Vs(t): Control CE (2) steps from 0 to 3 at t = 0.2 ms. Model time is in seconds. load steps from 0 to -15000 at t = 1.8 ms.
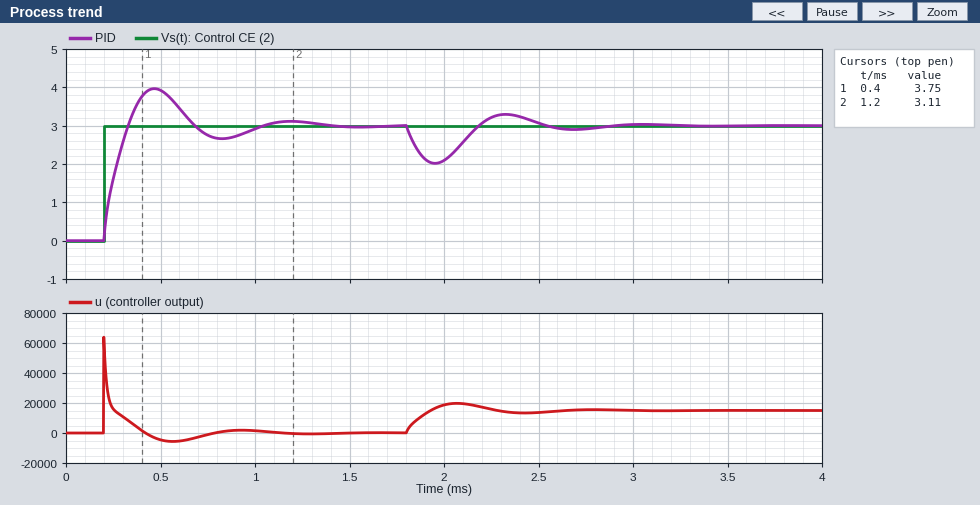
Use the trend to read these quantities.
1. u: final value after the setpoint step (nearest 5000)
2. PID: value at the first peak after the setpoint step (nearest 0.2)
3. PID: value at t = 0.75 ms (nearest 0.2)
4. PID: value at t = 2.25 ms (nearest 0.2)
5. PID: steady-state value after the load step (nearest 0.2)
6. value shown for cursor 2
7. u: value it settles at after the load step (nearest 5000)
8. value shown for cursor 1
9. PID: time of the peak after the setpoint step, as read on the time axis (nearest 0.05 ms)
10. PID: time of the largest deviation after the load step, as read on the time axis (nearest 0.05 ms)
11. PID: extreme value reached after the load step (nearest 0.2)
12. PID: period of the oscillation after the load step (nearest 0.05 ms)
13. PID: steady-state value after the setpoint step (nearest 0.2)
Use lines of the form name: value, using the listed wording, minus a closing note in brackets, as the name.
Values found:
u: final value after the setpoint step: 0
PID: value at the first peak after the setpoint step: 4.0
PID: value at t = 0.75 ms: 2.8
PID: value at t = 2.25 ms: 3.2
PID: steady-state value after the load step: 3.0
value shown for cursor 2: 3.11
u: value it settles at after the load step: 15000
value shown for cursor 1: 3.75
PID: time of the peak after the setpoint step, as read on the time axis: 0.45 ms
PID: time of the largest deviation after the load step, as read on the time axis: 1.95 ms
PID: extreme value reached after the load step: 2.0
PID: period of the oscillation after the load step: 0.75 ms
PID: steady-state value after the setpoint step: 3.0
